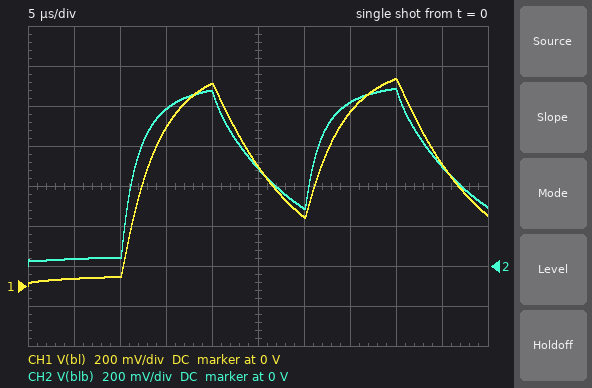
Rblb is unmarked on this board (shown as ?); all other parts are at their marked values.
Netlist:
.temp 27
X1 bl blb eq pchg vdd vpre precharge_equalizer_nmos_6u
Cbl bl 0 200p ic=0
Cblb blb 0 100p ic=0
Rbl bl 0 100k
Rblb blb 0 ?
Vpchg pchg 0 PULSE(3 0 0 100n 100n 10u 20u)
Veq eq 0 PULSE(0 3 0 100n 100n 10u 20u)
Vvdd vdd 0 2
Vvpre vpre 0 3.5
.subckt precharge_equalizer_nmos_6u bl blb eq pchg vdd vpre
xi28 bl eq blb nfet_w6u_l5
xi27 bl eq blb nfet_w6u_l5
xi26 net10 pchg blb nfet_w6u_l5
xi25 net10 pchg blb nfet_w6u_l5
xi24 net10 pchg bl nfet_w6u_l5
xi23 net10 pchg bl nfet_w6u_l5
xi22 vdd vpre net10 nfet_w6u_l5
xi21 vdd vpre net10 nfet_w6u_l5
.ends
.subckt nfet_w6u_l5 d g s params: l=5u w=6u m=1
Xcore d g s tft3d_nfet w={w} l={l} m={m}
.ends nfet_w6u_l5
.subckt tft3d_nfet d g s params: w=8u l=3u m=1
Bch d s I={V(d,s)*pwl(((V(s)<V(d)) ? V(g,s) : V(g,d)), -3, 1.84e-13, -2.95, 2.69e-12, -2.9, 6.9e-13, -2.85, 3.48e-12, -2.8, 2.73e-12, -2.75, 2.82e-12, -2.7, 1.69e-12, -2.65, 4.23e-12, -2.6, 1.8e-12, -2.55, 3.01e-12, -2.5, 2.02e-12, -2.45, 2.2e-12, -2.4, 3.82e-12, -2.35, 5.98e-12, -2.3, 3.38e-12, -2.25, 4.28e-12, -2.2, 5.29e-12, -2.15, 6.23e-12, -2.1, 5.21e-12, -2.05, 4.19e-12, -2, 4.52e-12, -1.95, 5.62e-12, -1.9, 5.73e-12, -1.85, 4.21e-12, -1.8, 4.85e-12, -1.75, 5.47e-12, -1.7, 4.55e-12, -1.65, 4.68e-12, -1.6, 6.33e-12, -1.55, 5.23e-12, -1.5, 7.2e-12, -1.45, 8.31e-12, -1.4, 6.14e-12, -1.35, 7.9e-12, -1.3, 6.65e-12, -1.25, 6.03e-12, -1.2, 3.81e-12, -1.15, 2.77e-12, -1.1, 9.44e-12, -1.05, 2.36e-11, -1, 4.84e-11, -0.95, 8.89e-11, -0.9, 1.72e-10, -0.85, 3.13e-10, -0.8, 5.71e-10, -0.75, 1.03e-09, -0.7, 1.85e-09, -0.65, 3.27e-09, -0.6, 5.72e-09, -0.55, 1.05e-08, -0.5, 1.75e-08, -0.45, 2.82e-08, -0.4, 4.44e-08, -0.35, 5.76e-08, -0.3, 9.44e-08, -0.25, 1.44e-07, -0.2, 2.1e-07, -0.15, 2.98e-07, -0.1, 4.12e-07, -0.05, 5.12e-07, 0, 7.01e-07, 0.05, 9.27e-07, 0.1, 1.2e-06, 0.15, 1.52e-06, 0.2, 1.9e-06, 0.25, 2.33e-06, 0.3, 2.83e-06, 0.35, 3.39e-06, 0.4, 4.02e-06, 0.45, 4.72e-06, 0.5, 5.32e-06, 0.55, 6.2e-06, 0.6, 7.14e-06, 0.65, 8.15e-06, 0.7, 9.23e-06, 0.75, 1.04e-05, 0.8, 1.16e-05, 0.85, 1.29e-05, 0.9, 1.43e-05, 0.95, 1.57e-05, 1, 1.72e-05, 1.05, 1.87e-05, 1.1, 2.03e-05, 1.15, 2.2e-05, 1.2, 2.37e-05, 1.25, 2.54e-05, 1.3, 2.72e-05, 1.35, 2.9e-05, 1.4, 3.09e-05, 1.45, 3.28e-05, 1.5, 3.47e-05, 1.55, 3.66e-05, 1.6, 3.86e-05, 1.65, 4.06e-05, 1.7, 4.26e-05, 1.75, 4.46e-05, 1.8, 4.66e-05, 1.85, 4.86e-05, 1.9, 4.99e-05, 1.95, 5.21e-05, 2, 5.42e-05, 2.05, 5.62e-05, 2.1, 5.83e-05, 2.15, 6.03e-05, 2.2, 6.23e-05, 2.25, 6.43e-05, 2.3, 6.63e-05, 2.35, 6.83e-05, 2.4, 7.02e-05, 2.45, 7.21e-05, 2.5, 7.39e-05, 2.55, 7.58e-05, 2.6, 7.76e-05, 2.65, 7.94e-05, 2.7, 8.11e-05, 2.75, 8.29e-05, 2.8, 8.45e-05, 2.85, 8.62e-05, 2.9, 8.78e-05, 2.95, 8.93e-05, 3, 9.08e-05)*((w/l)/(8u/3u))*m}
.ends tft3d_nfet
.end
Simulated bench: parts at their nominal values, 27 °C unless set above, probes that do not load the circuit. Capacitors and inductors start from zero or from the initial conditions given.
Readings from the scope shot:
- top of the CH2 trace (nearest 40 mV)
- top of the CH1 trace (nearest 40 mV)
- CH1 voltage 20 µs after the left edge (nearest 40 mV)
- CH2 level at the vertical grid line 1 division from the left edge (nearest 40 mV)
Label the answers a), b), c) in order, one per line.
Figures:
a) 880 mV
b) 1.04 V
c) 1.00 V
d) 40 mV
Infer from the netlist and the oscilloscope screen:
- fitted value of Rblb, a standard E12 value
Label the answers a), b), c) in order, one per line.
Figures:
a) 39 kΩ
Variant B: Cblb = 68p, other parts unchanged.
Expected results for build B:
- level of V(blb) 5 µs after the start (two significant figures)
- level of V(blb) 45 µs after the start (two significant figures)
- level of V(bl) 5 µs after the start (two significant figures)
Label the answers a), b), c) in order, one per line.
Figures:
a) 37 mV
b) 460 mV
c) 38 mV
